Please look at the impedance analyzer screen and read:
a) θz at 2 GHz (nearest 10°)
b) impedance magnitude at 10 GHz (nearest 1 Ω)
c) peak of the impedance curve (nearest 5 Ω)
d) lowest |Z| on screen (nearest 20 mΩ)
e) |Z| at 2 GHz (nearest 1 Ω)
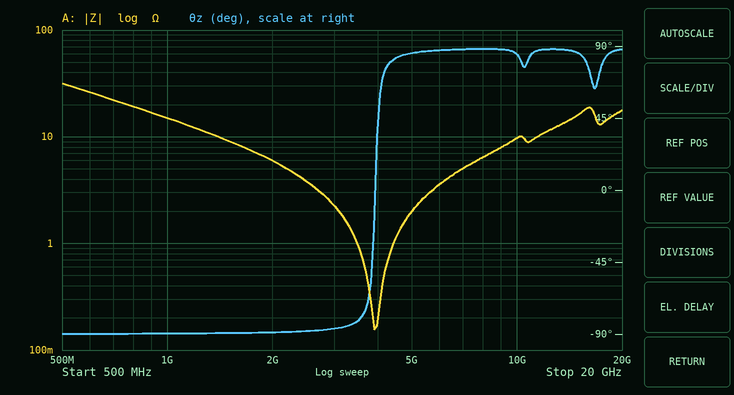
-90°
10 Ω
30 Ω
160 mΩ
6 Ω
